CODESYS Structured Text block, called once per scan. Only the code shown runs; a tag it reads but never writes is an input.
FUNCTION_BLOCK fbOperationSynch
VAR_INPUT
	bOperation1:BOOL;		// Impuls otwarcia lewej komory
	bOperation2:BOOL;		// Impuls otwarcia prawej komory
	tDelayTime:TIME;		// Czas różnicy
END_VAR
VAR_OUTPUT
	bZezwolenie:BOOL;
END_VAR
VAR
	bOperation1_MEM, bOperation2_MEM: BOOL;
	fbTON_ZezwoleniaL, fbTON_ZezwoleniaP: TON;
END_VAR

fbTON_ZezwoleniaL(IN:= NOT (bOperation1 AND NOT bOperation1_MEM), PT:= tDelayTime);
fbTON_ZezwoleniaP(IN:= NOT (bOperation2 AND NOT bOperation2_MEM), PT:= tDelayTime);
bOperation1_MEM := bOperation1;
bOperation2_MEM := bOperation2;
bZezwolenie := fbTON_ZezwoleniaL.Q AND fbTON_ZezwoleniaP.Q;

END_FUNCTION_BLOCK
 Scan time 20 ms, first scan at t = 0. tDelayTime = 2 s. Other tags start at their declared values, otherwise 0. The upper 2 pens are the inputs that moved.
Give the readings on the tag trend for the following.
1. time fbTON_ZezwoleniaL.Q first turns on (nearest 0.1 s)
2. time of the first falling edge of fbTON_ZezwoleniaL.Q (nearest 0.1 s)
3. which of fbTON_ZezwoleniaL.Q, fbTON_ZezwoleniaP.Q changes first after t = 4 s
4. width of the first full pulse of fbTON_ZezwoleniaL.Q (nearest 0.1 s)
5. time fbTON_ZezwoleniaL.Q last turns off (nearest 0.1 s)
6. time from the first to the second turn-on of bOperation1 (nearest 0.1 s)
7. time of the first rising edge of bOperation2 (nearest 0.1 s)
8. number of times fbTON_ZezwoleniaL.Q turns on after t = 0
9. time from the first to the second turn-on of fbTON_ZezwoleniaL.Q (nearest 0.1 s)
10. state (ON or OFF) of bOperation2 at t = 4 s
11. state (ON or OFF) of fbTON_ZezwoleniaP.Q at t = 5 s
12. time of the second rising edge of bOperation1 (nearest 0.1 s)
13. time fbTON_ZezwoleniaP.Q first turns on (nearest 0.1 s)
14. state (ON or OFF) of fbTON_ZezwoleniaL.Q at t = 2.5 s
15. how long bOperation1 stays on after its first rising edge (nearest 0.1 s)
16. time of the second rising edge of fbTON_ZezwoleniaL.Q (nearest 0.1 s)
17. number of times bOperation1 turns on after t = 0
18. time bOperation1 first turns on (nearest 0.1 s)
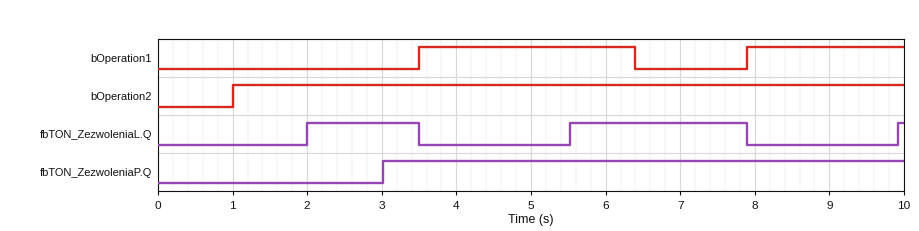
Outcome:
2.0 s
3.5 s
fbTON_ZezwoleniaL.Q
1.5 s
7.9 s
4.4 s
1.0 s
3
3.5 s
ON
ON
7.9 s
3.0 s
ON
2.9 s
5.5 s
2
3.5 s
